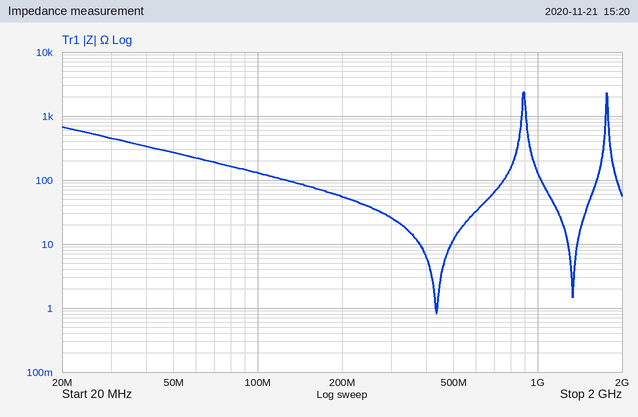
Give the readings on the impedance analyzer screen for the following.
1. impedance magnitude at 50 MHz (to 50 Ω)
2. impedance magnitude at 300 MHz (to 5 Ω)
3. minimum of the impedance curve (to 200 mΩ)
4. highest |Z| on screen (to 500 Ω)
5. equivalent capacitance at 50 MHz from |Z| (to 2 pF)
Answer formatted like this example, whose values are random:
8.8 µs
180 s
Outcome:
250 Ω
25 Ω
800 mΩ
2.5 kΩ
12 pF
